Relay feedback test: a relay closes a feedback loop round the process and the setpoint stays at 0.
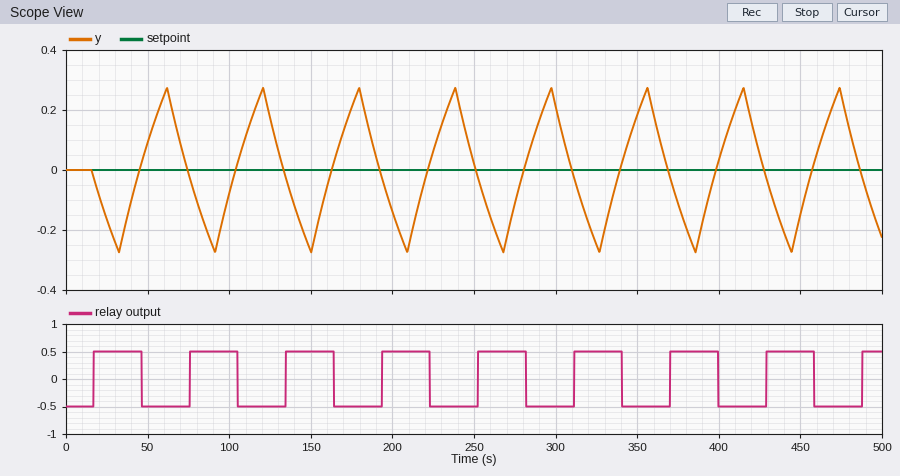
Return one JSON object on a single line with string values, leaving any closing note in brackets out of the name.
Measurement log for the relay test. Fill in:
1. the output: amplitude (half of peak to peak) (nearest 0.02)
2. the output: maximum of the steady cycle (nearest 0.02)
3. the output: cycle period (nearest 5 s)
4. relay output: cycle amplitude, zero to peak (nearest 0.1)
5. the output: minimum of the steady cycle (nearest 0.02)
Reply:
{"the output: amplitude (half of peak to peak)": "0.28", "the output: maximum of the steady cycle": "0.28", "the output: cycle period": "60 s", "relay output: cycle amplitude, zero to peak": "0.5", "the output: minimum of the steady cycle": "-0.28"}
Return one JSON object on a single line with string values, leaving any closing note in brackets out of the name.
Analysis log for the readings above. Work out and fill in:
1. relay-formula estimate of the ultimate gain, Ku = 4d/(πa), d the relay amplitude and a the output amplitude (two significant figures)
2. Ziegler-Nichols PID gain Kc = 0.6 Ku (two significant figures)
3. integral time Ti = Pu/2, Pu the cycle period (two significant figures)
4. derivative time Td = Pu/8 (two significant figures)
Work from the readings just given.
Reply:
{"relay-formula estimate of the ultimate gain, Ku = 4d/(πa), d the relay amplitude and a the output amplitude": "2.3", "Ziegler-Nichols PID gain Kc = 0.6 Ku": "1.4", "integral time Ti = Pu/2, Pu the cycle period": "30 s", "derivative time Td = Pu/8": "7.5 s"}
